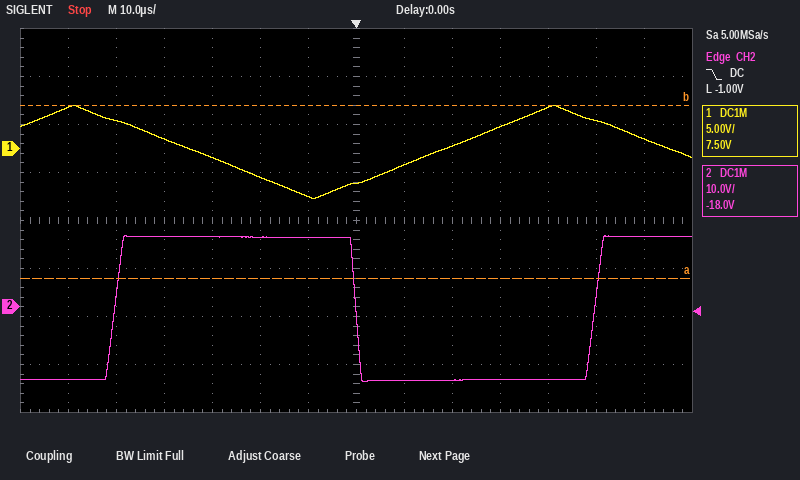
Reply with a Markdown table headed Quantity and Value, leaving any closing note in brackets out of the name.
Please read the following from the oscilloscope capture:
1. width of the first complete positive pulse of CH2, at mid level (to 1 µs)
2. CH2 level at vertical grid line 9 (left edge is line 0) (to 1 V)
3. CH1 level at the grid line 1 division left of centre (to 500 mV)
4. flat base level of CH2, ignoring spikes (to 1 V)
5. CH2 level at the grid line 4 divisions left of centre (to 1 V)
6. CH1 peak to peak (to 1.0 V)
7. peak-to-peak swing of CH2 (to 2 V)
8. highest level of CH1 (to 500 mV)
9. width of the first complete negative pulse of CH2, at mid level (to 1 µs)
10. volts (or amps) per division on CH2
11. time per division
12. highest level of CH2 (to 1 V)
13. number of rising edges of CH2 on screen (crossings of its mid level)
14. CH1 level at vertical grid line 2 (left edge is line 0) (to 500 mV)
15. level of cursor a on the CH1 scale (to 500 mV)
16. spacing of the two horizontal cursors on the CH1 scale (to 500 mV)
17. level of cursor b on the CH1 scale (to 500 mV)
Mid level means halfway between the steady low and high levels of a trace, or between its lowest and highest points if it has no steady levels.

| Quantity | Value |
|---|---|
| width of the first complete positive pulse of CH2, at mid level | 50 µs |
| CH2 level at vertical grid line 9 (left edge is line 0) | -15 V |
| CH1 level at the grid line 1 division left of centre | -5.0 V |
| flat base level of CH2, ignoring spikes | -15 V |
| CH2 level at the grid line 4 divisions left of centre | 15 V |
| CH1 peak to peak | 10.0 V |
| peak-to-peak swing of CH2 | 30 V |
| highest level of CH1 | 4.5 V |
| width of the first complete negative pulse of CH2, at mid level | 50 µs |
| volts (or amps) per division on CH2 | 10 V |
| time per division | 10 µs |
| highest level of CH2 | 15 V |
| number of rising edges of CH2 on screen | 2 |
| CH1 level at vertical grid line 2 (left edge is line 0) | 3.0 V |
| level of cursor a on the CH1 scale | -13.5 V |
| spacing of the two horizontal cursors on the CH1 scale | 18.0 V |
| level of cursor b on the CH1 scale | 4.5 V |
